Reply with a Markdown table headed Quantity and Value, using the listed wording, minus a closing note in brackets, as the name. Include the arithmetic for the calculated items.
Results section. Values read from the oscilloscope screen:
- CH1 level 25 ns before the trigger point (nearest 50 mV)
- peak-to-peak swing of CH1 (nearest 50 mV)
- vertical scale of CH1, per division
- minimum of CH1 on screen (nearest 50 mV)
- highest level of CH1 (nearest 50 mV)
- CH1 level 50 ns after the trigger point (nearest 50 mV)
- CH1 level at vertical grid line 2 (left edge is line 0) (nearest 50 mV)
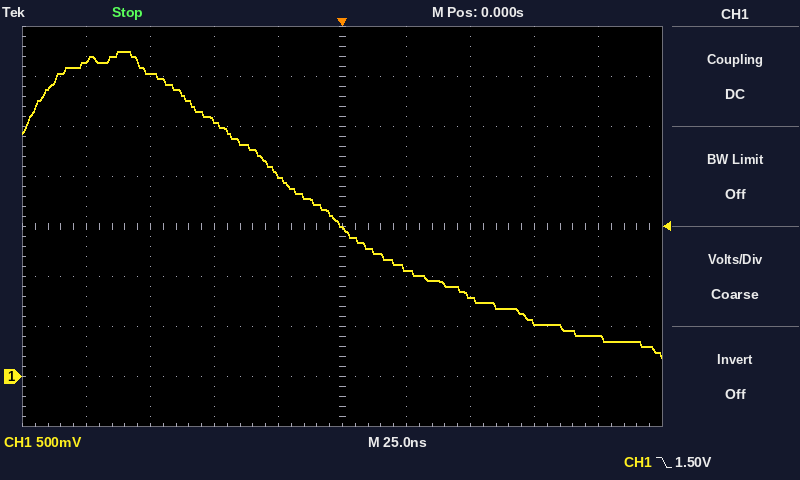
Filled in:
| Quantity | Value |
|---|---|
| CH1 level 25 ns before the trigger point | 2.00 V |
| peak-to-peak swing of CH1 | 3.25 V − (200 mV) = 3.05 V |
| vertical scale of CH1, per division | 500 mV |
| minimum of CH1 on screen | 200 mV |
| highest level of CH1 | 3.25 V |
| CH1 level 50 ns after the trigger point | 800 mV |
| CH1 level at vertical grid line 2 (left edge is line 0) | 3.05 V |
